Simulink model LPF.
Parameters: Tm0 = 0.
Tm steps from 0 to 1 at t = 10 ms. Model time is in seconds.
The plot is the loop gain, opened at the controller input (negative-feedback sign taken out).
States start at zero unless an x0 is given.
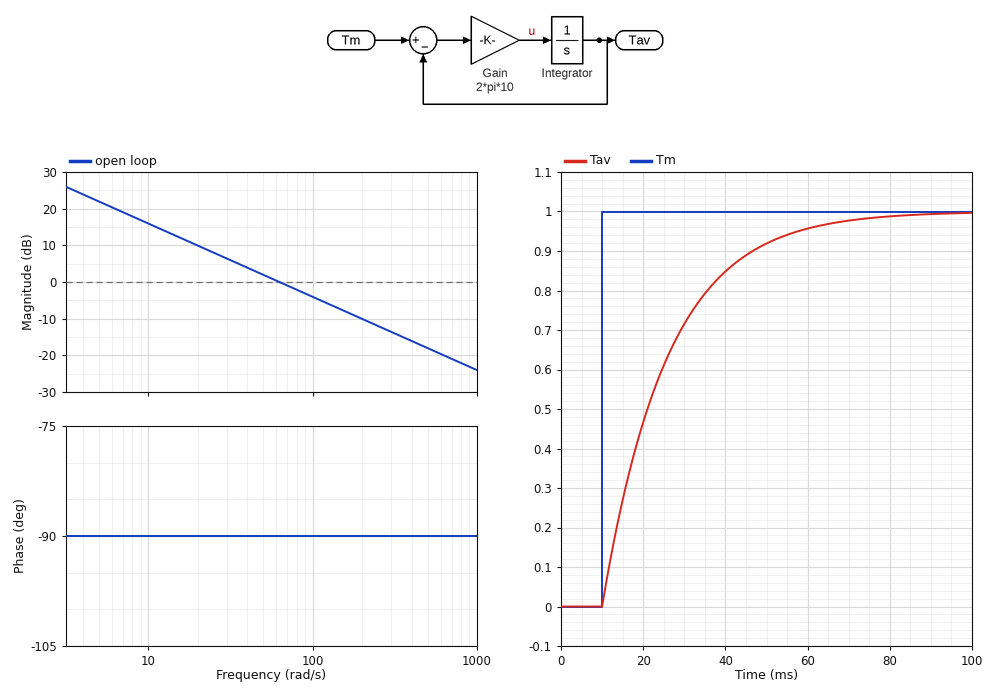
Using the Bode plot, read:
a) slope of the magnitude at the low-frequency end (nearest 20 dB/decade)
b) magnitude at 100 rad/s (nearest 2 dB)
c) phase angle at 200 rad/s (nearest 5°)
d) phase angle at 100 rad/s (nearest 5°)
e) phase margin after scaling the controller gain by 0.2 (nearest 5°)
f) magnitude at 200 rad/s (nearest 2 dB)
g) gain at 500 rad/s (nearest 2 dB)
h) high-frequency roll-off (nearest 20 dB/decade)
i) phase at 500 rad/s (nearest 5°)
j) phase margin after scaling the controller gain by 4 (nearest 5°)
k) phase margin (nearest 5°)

-20 dB/decade
-4 dB
-90°
-90°
90°
-10 dB
-18 dB
-20 dB/decade
-90°
90°
90°
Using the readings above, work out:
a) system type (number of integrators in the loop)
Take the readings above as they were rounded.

1
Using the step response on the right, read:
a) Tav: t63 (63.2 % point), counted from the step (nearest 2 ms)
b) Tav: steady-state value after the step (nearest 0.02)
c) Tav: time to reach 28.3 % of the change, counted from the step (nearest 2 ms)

16 ms
1.00
6 ms
